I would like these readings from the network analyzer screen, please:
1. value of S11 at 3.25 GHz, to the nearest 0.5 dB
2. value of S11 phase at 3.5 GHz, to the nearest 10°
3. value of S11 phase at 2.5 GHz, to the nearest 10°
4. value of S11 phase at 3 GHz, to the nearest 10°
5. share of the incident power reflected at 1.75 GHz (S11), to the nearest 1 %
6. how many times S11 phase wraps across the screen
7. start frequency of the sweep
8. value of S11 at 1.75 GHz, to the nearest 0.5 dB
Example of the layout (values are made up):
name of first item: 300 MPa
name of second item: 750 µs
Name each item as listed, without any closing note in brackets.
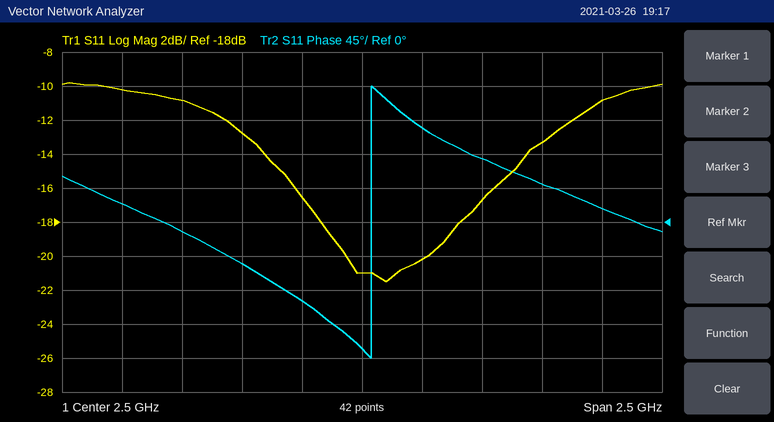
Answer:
value of S11 at 3.25 GHz, to the nearest 0.5 dB: -13.5 dB
value of S11 phase at 3.5 GHz, to the nearest 10°: 20°
value of S11 phase at 2.5 GHz, to the nearest 10°: -170°
value of S11 phase at 3 GHz, to the nearest 10°: 80°
share of the incident power reflected at 1.75 GHz (S11), to the nearest 1 %: 8 %
how many times S11 phase wraps across the screen: 1
start frequency of the sweep: 1.25 GHz
value of S11 at 1.75 GHz, to the nearest 0.5 dB: -11.0 dB
